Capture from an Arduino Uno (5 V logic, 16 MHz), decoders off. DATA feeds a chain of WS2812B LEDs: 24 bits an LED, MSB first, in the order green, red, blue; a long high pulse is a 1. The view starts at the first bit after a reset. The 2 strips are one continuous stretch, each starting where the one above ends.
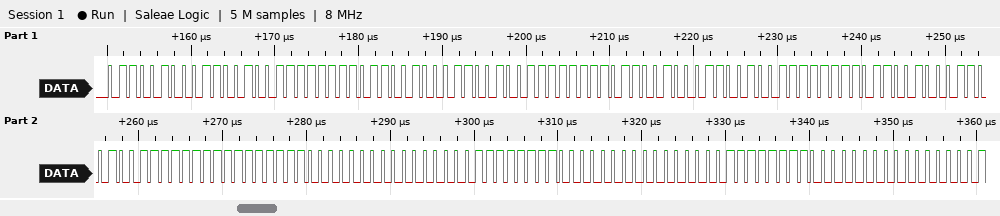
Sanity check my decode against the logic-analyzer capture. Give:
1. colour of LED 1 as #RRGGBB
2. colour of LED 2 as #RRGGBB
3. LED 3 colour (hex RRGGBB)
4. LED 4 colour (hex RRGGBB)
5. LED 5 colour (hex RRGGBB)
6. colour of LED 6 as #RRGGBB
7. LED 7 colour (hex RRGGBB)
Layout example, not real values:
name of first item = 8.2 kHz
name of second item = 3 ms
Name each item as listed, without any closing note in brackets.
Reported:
colour of LED 1 as #RRGGBB = #6464FF
colour of LED 2 as #RRGGBB = #6464FF
LED 3 colour = #6464FF
LED 4 colour = #6464FF
LED 5 colour = #00FF00
colour of LED 6 as #RRGGBB = #00FF00
LED 7 colour = #00FF00
